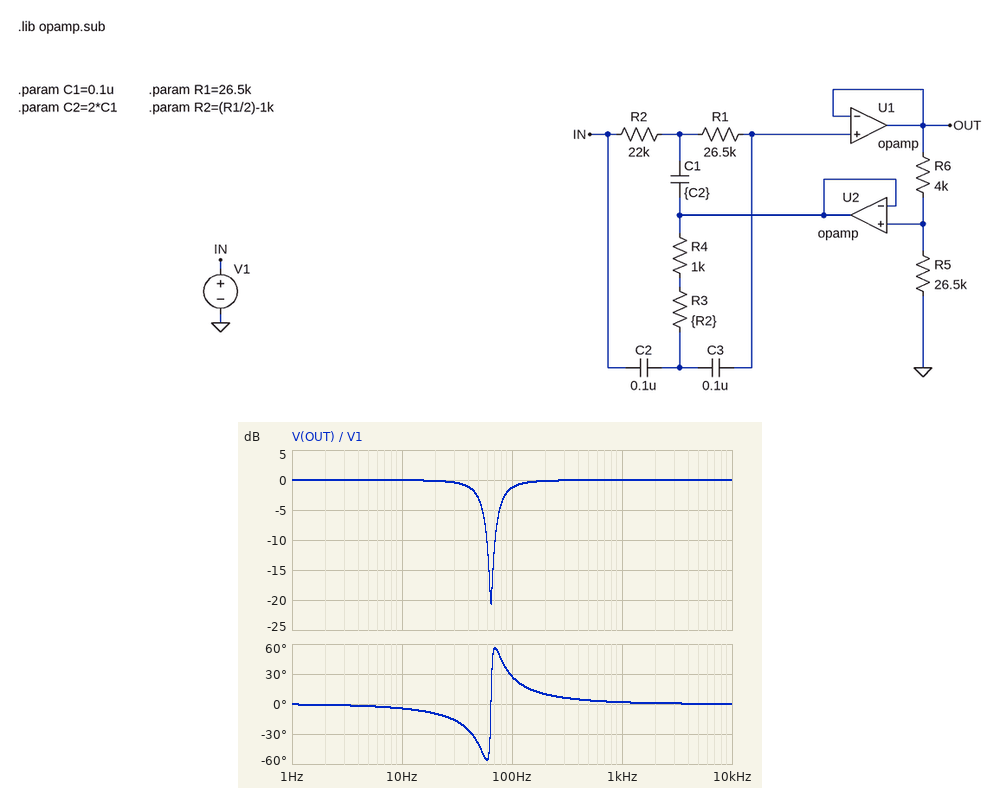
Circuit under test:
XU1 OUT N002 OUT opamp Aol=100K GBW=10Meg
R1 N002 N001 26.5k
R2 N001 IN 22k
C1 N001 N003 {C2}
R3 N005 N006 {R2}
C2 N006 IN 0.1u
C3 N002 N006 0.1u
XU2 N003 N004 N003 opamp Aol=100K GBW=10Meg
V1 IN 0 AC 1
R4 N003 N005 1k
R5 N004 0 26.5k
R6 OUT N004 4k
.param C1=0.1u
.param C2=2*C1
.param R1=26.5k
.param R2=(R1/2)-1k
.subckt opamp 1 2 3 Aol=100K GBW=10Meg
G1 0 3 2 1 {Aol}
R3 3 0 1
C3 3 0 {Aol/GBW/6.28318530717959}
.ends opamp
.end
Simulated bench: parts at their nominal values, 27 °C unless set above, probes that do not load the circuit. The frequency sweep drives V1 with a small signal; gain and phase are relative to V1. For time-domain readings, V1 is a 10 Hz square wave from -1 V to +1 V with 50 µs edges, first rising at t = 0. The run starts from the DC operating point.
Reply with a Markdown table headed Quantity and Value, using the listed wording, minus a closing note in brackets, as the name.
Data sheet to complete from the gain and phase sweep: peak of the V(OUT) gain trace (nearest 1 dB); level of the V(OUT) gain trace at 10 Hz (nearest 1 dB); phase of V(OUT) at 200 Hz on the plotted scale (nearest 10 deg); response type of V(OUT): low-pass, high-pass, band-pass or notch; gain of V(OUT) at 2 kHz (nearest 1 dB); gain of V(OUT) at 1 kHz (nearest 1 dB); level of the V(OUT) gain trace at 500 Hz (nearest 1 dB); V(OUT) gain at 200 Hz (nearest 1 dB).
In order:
| Quantity | Value |
|---|---|
| peak of the V(OUT) gain trace | 0 dB |
| level of the V(OUT) gain trace at 10 Hz | 0 dB |
| phase of V(OUT) at 200 Hz on the plotted scale | 10 deg |
| response type of V(OUT): low-pass, high-pass, band-pass or notch | notch |
| gain of V(OUT) at 2 kHz | 0 dB |
| gain of V(OUT) at 1 kHz | 0 dB |
| level of the V(OUT) gain trace at 500 Hz | 0 dB |
| V(OUT) gain at 200 Hz | 0 dB |
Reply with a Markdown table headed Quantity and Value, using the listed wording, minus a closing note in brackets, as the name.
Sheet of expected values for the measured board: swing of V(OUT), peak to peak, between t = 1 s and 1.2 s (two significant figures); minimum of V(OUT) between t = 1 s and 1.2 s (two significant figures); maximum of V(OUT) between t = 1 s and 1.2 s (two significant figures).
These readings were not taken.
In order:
| Quantity | Value |
|---|---|
| swing of V(OUT), peak to peak, between t = 1 s and 1.2 s | 2.6 V |
| minimum of V(OUT) between t = 1 s and 1.2 s | -1.3 V |
| maximum of V(OUT) between t = 1 s and 1.2 s | 1.3 V |
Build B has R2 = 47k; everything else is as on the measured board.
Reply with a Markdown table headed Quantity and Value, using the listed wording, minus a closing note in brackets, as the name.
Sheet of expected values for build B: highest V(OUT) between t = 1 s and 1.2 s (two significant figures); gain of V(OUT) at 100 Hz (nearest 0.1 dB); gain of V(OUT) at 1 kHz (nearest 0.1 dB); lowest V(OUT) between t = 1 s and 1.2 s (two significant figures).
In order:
| Quantity | Value |
|---|---|
| highest V(OUT) between t = 1 s and 1.2 s | 1.4 V |
| gain of V(OUT) at 100 Hz | -0.4 dB |
| gain of V(OUT) at 1 kHz | 0 dB |
| lowest V(OUT) between t = 1 s and 1.2 s | -1.4 V |
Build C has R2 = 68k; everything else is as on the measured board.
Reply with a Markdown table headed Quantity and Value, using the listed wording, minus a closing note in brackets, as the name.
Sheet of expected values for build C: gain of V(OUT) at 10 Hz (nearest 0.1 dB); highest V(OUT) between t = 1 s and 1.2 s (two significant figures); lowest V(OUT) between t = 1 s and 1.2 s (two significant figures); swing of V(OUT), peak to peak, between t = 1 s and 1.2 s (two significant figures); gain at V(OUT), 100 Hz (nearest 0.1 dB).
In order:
| Quantity | Value |
|---|---|
| gain of V(OUT) at 10 Hz | -0.1 dB |
| highest V(OUT) between t = 1 s and 1.2 s | 1.4 V |
| lowest V(OUT) between t = 1 s and 1.2 s | -1.4 V |
| swing of V(OUT), peak to peak, between t = 1 s and 1.2 s | 2.7 V |
| gain at V(OUT), 100 Hz | -0.3 dB |
